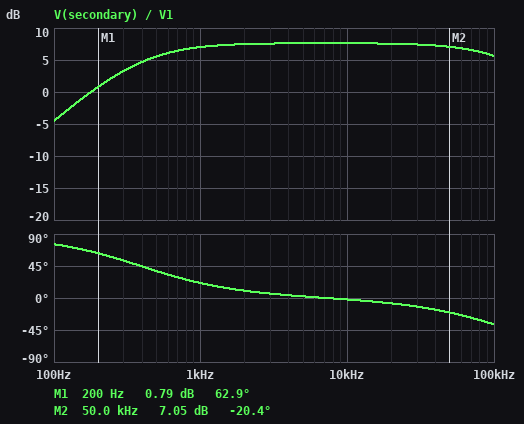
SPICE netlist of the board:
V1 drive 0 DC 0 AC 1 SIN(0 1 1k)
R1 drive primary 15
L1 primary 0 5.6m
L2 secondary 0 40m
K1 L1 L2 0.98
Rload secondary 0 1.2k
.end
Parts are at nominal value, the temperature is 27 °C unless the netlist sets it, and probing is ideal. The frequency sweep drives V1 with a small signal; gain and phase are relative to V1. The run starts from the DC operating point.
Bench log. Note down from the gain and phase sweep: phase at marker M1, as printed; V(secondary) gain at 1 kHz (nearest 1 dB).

62.9 deg
7 dB
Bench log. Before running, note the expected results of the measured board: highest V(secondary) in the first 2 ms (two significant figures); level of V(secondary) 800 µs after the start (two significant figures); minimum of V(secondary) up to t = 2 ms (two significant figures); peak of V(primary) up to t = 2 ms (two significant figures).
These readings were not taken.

2.2 V
-1.9 V
-2.4 V
840 mV
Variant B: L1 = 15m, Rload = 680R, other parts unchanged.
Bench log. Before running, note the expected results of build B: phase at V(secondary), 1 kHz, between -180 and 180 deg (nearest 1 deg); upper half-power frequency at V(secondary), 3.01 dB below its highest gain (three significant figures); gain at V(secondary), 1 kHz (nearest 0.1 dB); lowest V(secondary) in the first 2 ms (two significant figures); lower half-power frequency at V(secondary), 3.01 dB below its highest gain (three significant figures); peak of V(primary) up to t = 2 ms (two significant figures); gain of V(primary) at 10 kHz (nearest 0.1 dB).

8 deg
72.5 kHz
3.5 dB
-1.6 V
150 Hz
890 mV
-0.5 dB
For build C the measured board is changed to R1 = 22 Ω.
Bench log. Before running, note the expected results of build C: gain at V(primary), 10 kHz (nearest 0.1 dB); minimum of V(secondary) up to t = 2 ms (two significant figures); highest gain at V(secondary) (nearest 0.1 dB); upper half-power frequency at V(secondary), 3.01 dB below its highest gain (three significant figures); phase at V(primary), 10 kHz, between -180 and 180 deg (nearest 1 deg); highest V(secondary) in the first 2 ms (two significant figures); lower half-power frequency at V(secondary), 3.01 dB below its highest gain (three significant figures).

-1.0 dB
-2.1 V
7.3 dB
137 kHz
4 deg
2.0 V
551 Hz
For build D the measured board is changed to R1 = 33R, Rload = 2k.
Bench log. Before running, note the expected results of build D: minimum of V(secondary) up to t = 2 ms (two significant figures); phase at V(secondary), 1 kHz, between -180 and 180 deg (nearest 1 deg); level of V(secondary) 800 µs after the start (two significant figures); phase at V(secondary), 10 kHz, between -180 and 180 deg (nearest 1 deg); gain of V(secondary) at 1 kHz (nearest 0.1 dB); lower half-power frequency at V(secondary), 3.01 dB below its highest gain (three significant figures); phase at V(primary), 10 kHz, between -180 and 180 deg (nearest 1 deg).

-1.8 V
40 deg
-970 mV
2 deg
5.1 dB
836 Hz
5 deg
